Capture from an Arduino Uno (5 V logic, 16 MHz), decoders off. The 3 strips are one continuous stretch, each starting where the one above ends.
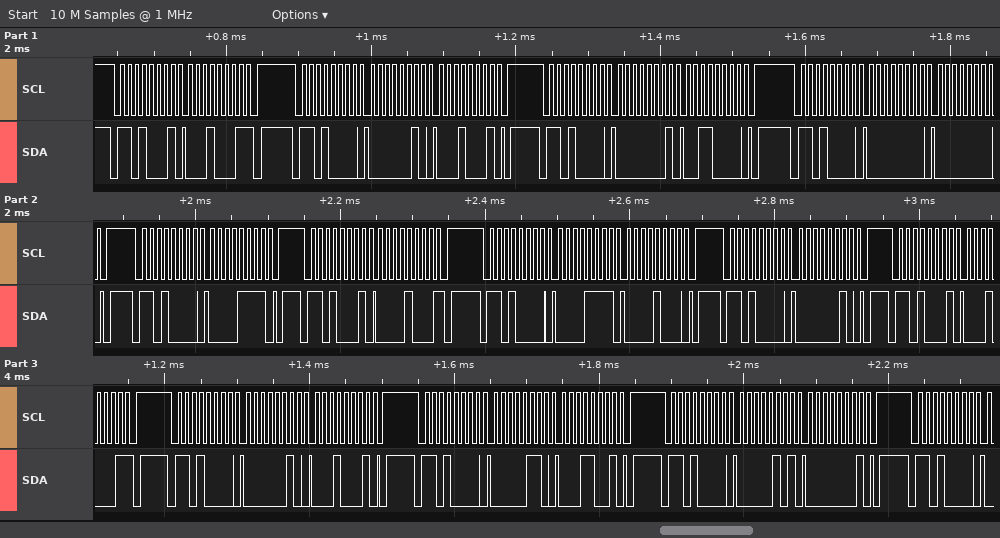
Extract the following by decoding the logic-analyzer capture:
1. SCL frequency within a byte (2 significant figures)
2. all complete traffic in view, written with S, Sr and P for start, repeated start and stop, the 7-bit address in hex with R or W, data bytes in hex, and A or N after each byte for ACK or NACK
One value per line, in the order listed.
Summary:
100 kHz
S 68R A 11 N P S 68W A 02 A 11 A P S 68W A 01 A 30 A P S 68W A 00 A 00 A P S 68W A 0F A P S 68R A 08 N P S 68W A 0F A 08 A P S 68W A 02 A P S 68R A 11 N P S 68W A 02 A 11 A P S 68W A 06 A 19 A P S 68W A 05 A 01 A P S 68W A
